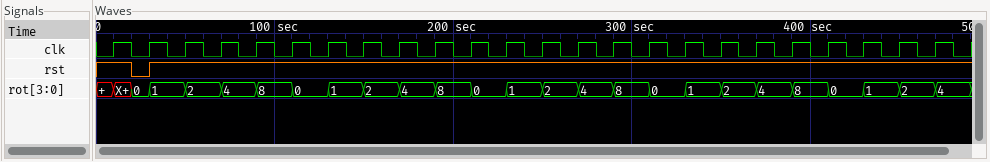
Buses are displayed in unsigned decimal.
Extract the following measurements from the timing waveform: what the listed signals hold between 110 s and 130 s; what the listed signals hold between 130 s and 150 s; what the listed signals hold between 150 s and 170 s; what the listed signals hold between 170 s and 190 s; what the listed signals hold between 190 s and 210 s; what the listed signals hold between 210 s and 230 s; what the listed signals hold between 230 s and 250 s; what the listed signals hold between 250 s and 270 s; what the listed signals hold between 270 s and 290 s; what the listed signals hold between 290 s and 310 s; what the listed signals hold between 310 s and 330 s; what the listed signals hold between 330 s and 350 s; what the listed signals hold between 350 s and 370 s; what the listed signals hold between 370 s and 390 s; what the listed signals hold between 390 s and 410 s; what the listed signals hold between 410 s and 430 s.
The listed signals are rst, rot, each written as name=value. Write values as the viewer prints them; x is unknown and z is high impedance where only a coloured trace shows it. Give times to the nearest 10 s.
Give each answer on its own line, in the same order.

rst=1, rot=0
rst=1, rot=1
rst=1, rot=2
rst=1, rot=4
rst=1, rot=8
rst=1, rot=0
rst=1, rot=1
rst=1, rot=2
rst=1, rot=4
rst=1, rot=8
rst=1, rot=0
rst=1, rot=1
rst=1, rot=2
rst=1, rot=4
rst=1, rot=8
rst=1, rot=0
